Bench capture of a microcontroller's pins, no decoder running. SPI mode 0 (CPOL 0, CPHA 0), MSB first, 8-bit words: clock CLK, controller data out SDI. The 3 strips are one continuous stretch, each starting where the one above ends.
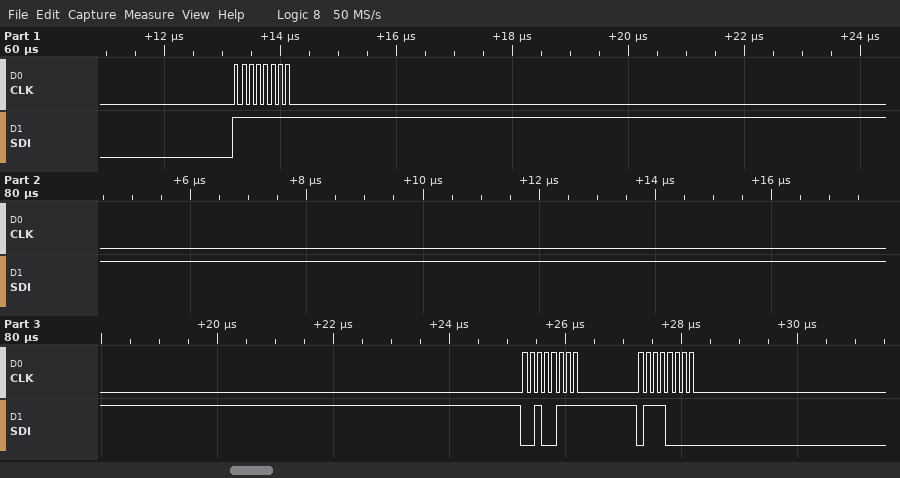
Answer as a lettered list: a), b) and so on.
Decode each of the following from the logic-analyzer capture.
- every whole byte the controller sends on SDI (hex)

a) FF 27 70
